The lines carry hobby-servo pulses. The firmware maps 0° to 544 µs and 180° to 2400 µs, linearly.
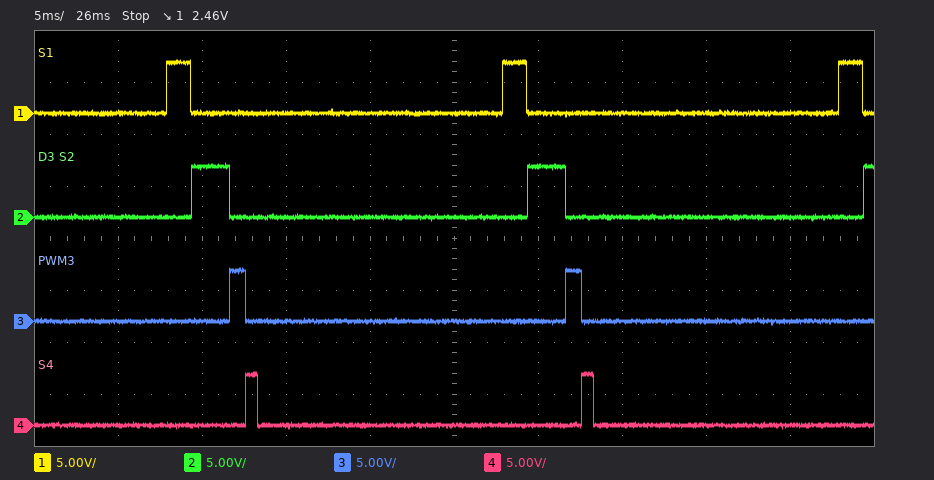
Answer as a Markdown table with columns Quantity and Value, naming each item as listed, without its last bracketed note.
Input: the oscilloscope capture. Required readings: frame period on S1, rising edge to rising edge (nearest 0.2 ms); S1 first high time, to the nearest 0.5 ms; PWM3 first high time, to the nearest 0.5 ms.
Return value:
| Quantity | Value |
|---|---|
| frame period on S1, rising edge to rising edge | 20.0 ms |
| S1 first high time, to the nearest 0.5 ms | 1.5 ms |
| PWM3 first high time, to the nearest 0.5 ms | 1.0 ms |
